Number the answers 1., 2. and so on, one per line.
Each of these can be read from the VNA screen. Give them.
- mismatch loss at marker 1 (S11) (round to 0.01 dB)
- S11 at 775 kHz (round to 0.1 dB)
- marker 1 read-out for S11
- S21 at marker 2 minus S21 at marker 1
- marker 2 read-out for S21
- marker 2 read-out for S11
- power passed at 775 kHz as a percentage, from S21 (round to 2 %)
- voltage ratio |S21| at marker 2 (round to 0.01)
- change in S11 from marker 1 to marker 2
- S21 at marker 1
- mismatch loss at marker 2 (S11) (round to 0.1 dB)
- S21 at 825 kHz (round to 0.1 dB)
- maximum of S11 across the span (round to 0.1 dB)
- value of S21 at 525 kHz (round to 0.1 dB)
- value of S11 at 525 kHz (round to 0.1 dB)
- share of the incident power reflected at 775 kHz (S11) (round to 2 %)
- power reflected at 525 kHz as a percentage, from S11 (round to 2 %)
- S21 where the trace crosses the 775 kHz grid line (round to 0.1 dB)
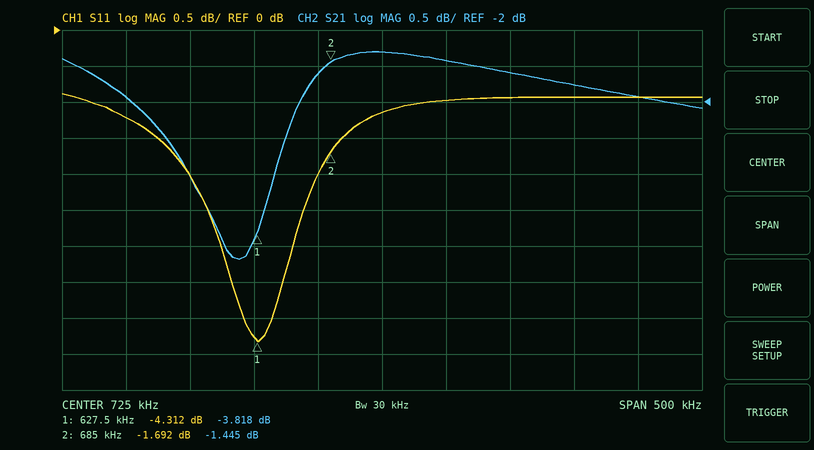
1. 2.01 dB
2. -1.0 dB
3. -4.312 dB
4. 2.373 dB
5. -1.445 dB
6. -1.692 dB
7. 72 %
8. 0.85
9. 2.620 dB
10. -3.818 dB
11. 4.9 dB
12. -1.6 dB
13. -0.9 dB
14. -1.9 dB
15. -1.2 dB
16. 80 %
17. 76 %
18. -1.4 dB
